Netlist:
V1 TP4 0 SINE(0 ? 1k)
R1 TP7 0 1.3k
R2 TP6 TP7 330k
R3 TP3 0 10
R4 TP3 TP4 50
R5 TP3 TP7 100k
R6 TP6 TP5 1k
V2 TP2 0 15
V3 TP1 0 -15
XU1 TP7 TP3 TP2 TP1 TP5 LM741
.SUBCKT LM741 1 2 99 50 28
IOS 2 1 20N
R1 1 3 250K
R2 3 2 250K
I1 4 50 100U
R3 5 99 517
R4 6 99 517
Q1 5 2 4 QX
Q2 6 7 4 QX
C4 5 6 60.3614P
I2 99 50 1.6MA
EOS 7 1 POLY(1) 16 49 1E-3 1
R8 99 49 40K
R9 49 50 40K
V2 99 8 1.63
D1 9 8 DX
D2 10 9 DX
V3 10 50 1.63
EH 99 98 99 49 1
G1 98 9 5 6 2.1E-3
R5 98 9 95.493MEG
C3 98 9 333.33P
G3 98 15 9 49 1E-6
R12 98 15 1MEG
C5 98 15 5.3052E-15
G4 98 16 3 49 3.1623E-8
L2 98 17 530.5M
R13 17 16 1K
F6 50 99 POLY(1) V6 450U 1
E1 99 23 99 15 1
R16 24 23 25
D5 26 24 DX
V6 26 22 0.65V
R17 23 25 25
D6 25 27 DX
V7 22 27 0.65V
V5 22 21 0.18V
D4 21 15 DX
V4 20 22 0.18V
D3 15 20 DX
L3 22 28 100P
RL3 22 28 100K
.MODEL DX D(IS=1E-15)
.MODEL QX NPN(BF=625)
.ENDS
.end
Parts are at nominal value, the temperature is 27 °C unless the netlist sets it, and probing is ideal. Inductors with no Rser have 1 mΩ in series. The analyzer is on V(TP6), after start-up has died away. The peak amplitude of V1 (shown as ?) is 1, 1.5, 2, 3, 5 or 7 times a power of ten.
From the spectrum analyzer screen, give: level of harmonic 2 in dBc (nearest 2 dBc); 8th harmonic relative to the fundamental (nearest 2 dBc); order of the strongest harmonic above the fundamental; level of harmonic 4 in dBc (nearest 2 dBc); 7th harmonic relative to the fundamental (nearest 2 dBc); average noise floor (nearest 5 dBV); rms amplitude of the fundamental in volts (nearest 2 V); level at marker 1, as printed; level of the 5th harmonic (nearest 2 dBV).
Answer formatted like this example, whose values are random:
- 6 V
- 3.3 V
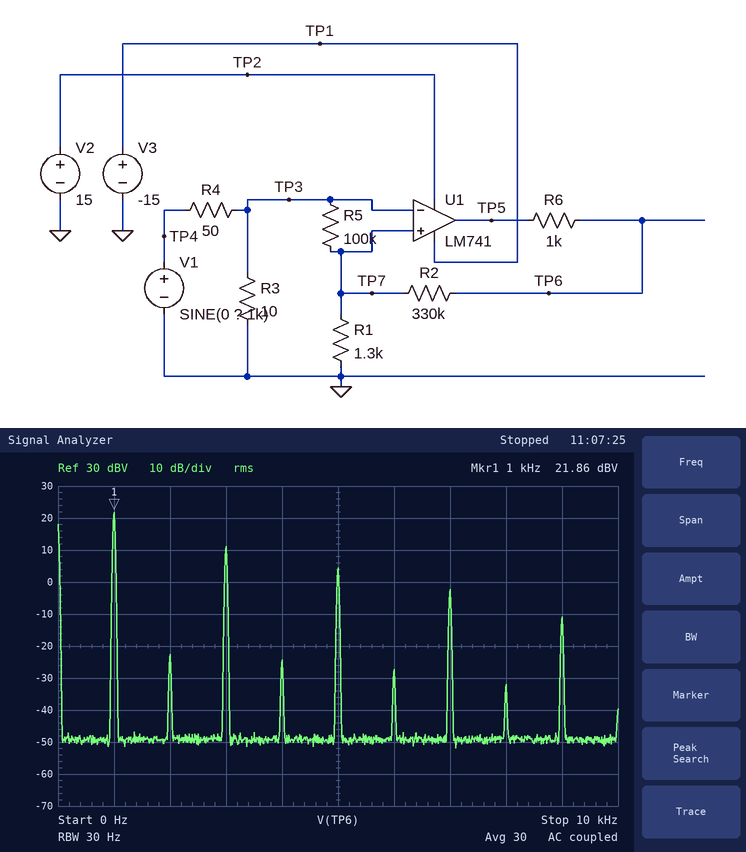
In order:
- -44 dBc
- -54 dBc
- 3
- -46 dBc
- -24 dBc
- -50 dBV
- 12 V
- 21.86 dBV
- 4 dBV
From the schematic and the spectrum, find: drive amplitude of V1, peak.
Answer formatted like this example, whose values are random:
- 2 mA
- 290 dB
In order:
- 1 V
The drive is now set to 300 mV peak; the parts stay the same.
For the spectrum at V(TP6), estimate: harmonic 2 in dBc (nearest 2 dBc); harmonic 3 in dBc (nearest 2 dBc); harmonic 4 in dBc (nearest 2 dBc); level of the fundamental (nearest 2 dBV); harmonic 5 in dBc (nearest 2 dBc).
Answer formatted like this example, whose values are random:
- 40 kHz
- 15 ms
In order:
- -6 dBc
- -12 dBc
- -18 dBc
- -34 dBV
- -24 dBc
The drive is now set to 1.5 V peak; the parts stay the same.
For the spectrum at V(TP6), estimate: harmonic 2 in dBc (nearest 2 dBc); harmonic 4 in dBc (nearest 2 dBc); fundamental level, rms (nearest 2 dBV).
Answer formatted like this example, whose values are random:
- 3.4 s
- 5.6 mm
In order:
- -48 dBc
- -50 dBc
- 22 dBV
